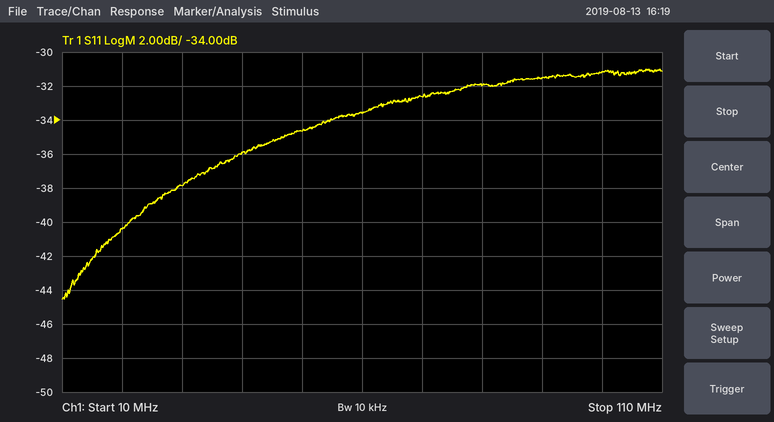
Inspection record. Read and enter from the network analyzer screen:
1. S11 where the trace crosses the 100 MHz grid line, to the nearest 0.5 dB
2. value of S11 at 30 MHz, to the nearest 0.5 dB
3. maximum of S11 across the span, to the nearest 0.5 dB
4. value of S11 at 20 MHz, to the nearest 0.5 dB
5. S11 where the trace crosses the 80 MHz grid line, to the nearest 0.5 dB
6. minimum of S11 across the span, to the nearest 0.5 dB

-31.0 dB
-38.0 dB
-31.0 dB
-40.5 dB
-32.0 dB
-44.5 dB
